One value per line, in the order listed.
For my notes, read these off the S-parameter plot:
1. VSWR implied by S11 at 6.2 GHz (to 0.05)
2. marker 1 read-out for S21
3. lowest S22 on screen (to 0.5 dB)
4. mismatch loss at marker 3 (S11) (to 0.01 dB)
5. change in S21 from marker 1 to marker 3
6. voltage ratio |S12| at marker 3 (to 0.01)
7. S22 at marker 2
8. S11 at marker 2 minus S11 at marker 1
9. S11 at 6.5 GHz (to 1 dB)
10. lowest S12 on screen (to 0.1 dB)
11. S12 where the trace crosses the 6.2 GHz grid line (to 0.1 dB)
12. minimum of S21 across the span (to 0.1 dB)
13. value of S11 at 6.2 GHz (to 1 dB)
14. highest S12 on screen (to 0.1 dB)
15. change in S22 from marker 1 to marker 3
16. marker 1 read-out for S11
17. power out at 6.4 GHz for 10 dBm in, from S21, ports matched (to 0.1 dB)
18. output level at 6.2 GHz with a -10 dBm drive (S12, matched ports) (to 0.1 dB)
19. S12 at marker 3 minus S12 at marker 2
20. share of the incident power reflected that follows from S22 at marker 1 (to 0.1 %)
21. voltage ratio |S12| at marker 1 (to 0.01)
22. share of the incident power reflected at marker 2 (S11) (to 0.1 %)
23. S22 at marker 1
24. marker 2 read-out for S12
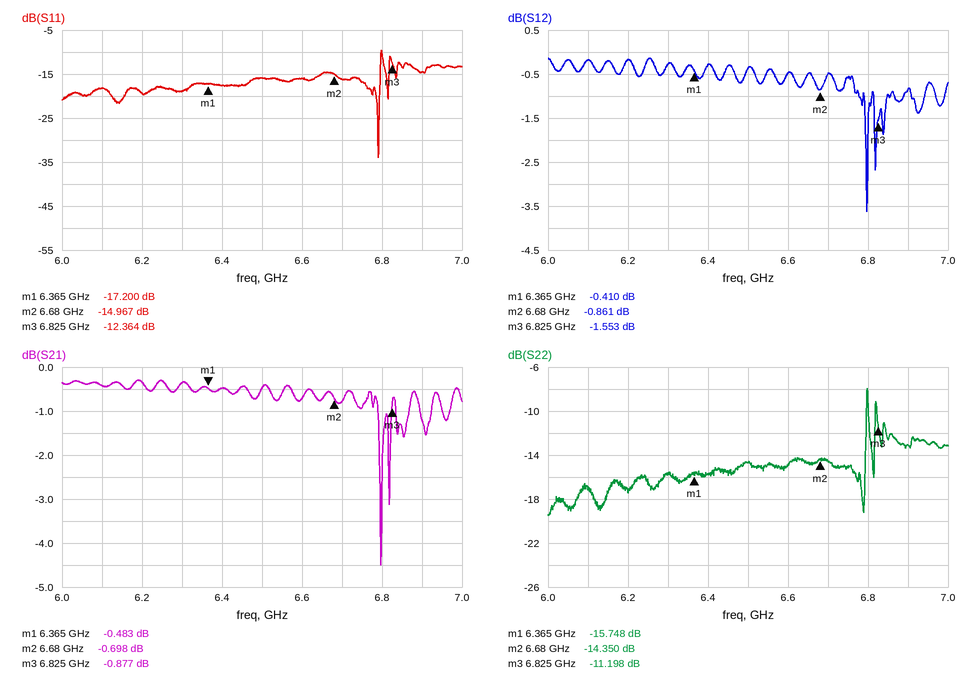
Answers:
1.25
-0.483 dB
-19.5 dB
0.26 dB
-0.394 dB
0.84
-14.350 dB
2.233 dB
-16 dB
-3.6 dB
-0.2 dB
-4.5 dB
-19 dB
-0.1 dB
4.550 dB
-17.200 dB
9.5 dBm
-10.2 dBm
-0.692 dB
2.7 %
0.95
3.2 %
-15.748 dB
-0.861 dB
